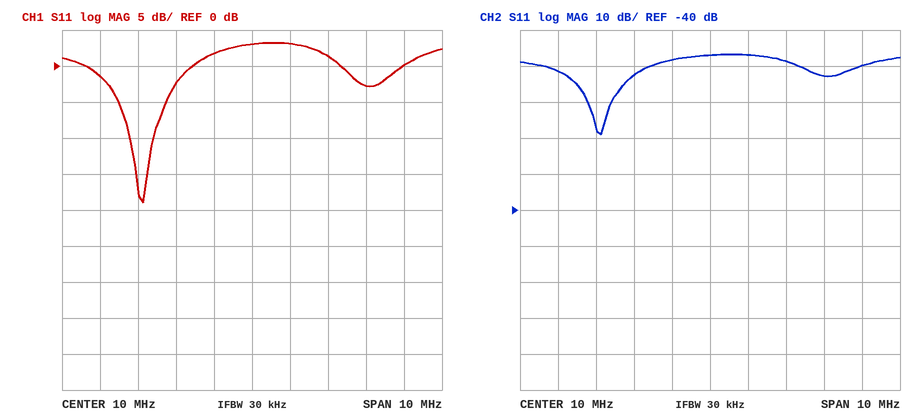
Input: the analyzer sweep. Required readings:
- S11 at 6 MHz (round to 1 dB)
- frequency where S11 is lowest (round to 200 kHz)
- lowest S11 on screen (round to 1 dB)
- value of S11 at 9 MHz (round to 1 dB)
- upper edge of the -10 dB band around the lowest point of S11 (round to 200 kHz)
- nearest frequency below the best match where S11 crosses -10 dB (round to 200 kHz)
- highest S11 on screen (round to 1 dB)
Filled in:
-1 dB
7.2 MHz
-19 dB
2 dB
7.4 MHz
6.8 MHz
3 dB
